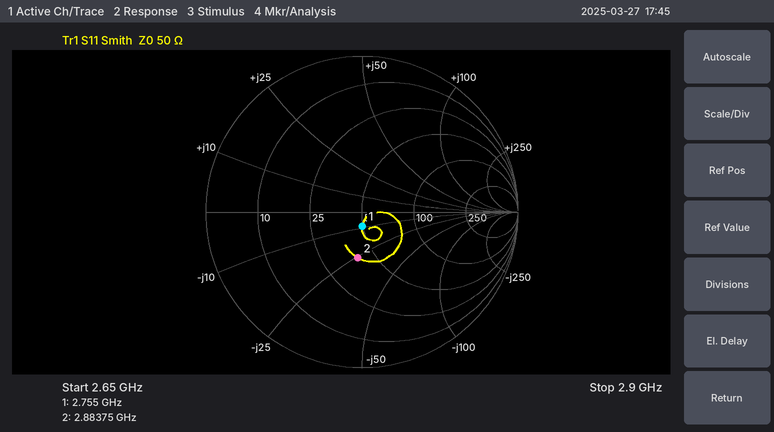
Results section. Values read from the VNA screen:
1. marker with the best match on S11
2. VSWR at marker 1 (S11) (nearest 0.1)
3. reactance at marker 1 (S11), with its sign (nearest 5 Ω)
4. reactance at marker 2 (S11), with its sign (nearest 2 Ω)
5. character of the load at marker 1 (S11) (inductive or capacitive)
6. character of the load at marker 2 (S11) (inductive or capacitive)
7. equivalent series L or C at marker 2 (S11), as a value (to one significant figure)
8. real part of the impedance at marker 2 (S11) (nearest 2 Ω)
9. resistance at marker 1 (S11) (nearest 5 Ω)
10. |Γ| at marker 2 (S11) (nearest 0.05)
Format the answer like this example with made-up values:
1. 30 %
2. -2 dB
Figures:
1. marker 1
2. 1.2
3. -10 Ω
4. -26 Ω
5. capacitive
6. capacitive
7. 2 pF
8. 40 Ω
9. 50 Ω
10. 0.30
